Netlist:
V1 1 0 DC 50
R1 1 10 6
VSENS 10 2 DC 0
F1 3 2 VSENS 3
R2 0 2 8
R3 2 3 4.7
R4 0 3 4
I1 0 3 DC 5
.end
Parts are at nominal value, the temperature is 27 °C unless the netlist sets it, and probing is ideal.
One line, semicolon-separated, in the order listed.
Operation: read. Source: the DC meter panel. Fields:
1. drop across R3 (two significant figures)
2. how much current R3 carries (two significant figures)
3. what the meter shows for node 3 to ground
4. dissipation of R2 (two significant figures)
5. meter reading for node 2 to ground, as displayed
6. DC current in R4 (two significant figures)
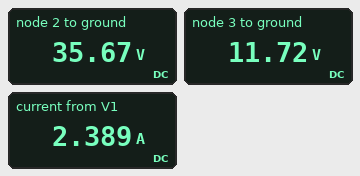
24 V; 5.1 A; 11.72 V; 160 W; 35.67 V; 2.9 A
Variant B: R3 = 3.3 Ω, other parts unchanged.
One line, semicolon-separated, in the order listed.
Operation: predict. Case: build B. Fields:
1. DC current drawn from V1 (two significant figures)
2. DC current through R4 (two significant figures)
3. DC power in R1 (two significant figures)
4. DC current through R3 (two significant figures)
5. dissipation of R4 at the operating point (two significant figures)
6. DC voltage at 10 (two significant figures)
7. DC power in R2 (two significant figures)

2.6 A; 3.4 A; 42 W; 6.3 A; 45 W; 34 V; 150 W
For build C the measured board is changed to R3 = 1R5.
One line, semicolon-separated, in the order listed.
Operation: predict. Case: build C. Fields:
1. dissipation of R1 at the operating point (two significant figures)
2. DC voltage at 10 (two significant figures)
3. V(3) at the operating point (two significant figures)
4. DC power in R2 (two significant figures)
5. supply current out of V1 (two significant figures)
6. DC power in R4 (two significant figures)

61 W; 31 V; 17 V; 120 W; 3.2 A; 76 W
